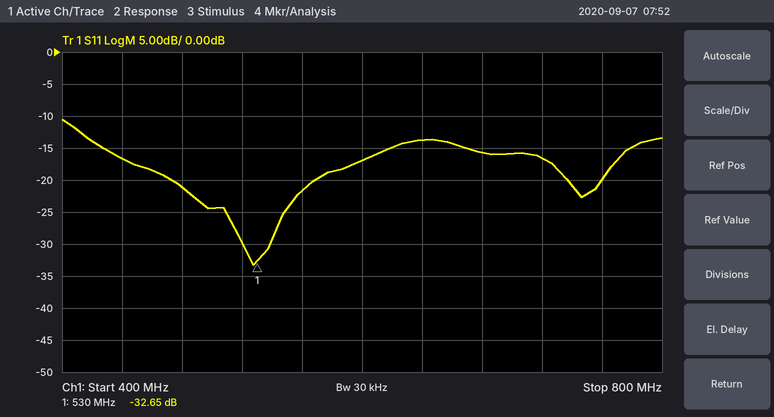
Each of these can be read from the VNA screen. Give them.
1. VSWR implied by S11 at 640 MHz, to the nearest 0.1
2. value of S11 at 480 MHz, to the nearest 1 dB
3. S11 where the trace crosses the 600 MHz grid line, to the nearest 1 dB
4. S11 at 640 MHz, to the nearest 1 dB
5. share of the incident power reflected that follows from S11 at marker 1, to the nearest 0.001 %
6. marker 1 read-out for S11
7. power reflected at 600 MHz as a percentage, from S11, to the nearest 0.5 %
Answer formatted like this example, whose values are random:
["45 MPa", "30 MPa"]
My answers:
["1.5", "-21 dB", "-17 dB", "-14 dB", "0.054 %", "-32.65 dB", "2.0 %"]
